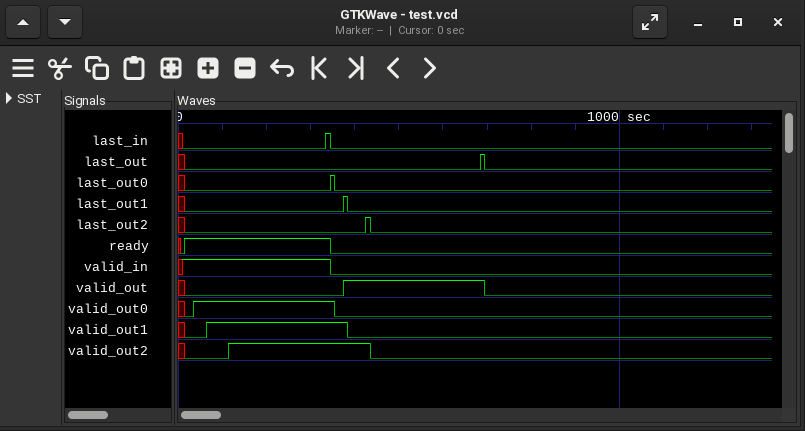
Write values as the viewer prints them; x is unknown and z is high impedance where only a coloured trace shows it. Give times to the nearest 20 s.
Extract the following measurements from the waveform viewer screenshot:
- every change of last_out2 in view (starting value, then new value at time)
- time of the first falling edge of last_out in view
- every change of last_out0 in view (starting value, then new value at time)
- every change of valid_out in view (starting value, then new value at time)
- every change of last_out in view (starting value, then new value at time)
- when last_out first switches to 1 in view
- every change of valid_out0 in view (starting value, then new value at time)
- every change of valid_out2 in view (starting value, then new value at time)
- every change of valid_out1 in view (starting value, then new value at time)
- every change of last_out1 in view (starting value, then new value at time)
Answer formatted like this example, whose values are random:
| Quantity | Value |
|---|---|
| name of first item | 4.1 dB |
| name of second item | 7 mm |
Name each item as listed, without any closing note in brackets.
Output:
| Quantity | Value |
|---|---|
| every change of last_out2 in view | x, 0 at 20 s, 1 at 420 s, 0 at 440 s |
| time of the first falling edge of last_out in view | 700 s |
| every change of last_out0 in view | x, 0 at 20 s, 1 at 340 s, 0 at 360 s |
| every change of valid_out in view | x, 0 at 20 s, 1 at 380 s, 0 at 700 s |
| every change of last_out in view | x, 0 at 20 s, 1 at 680 s, 0 at 700 s |
| when last_out first switches to 1 in view | 680 s |
| every change of valid_out0 in view | x, 0 at 20 s, 1 at 40 s, 0 at 360 s |
| every change of valid_out2 in view | x, 0 at 20 s, 1 at 120 s, 0 at 440 s |
| every change of valid_out1 in view | x, 0 at 20 s, 1 at 60 s, 0 at 380 s |
| every change of last_out1 in view | x, 0 at 20 s, 1 at 380 s, 0 at 380 s |
